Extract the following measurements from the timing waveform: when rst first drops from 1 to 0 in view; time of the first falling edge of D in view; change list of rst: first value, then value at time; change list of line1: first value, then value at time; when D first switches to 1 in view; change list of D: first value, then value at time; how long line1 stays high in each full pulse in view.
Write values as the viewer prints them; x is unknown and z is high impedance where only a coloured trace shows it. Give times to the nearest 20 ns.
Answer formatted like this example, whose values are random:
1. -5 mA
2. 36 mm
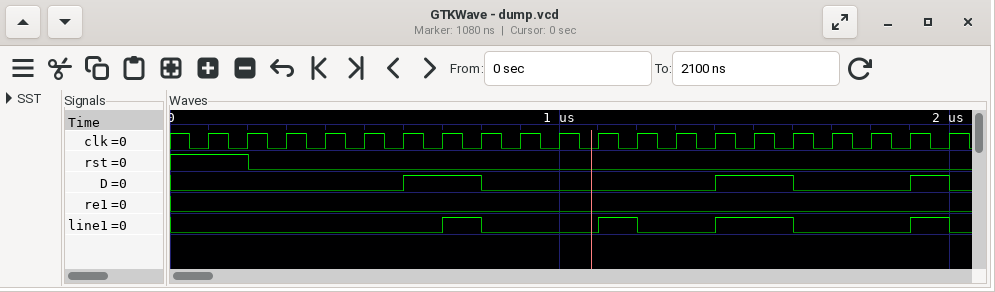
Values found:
1. 200 ns
2. 800 ns
3. 1, 0 at 200 ns
4. 0, 1 at 700 ns, 0 at 800 ns, 1 at 1100 ns, 0 at 1200 ns, 1 at 1400 ns, 0 at 1600 ns, 1 at 1900 ns, 0 at 2000 ns
5. 600 ns
6. 0, 1 at 600 ns, 0 at 800 ns, 1 at 1400 ns, 0 at 1600 ns, 1 at 1900 ns, 0 at 2000 ns
7. 100 ns, 100 ns, 200 ns, 100 ns
